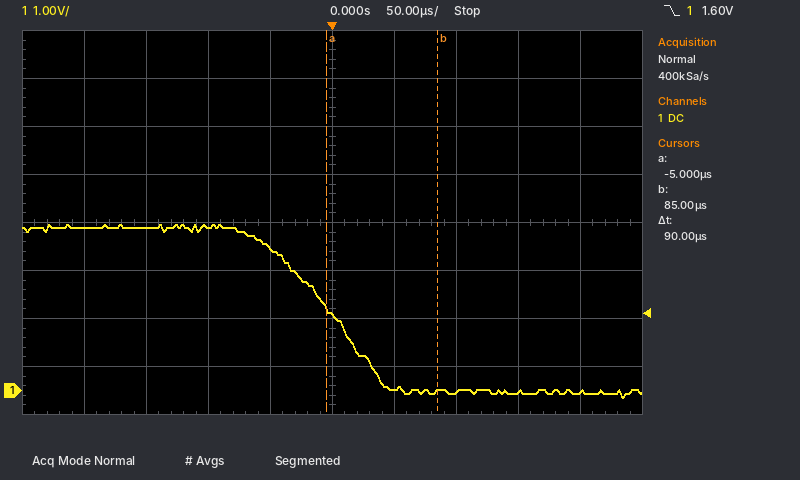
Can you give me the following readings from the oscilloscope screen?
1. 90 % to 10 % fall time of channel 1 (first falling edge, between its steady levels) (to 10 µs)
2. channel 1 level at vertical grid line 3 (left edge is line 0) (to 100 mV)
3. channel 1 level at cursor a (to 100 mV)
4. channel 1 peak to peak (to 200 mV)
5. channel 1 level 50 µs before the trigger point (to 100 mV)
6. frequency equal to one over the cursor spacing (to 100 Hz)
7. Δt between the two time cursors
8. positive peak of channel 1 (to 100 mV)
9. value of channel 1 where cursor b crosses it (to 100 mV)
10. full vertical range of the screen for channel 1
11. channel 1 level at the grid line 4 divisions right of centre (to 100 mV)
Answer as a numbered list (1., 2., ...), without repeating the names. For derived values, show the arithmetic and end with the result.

1. 90 µs
2. 3.4 V
3. 1.7 V
4. 3.6 V
5. 3.0 V
6. 1 / 90 µs ≈ 11.1 kHz
7. 90 µs
8. 3.5 V
9. 0.0 V
10. 8 V
11. 0.0 V
